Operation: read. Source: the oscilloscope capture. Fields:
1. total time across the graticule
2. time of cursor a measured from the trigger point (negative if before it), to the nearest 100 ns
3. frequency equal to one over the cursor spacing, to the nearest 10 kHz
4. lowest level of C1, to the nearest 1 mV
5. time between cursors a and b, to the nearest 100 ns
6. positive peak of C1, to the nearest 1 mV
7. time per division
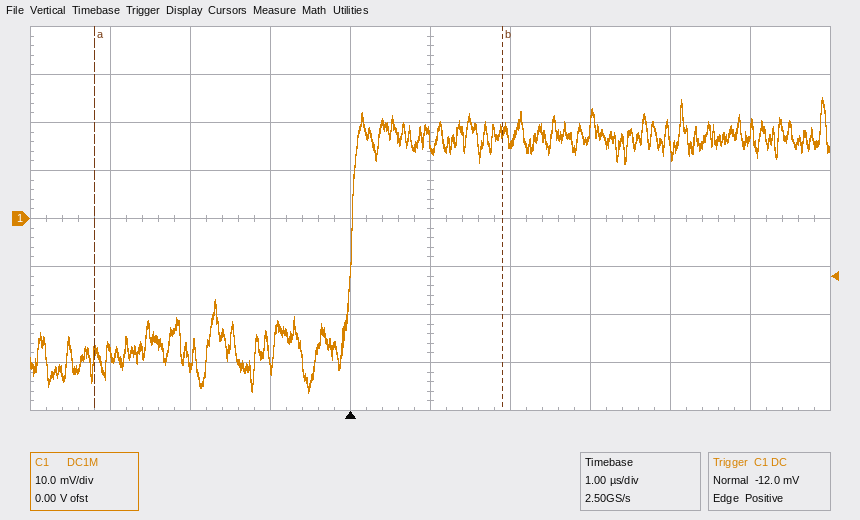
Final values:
10 µs
-3.2 µs
200 kHz
-36 mV
5.1 µs
25 mV
1 µs
